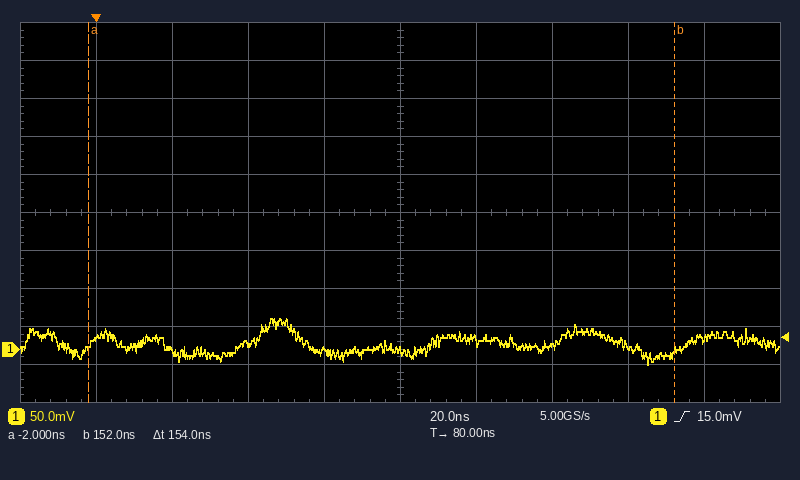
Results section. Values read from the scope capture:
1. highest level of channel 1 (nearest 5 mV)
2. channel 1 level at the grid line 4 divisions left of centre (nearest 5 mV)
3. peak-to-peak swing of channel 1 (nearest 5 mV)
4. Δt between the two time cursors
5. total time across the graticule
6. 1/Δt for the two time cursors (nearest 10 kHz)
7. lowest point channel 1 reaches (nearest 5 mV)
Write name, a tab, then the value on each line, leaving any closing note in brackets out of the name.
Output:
highest level of channel 1	40 mV
channel 1 level at the grid line 4 divisions left of centre	15 mV
peak-to-peak swing of channel 1	60 mV
Δt between the two time cursors	154 ns
total time across the graticule	200 ns
1/Δt for the two time cursors	6.49 MHz
lowest point channel 1 reaches	-20 mV
